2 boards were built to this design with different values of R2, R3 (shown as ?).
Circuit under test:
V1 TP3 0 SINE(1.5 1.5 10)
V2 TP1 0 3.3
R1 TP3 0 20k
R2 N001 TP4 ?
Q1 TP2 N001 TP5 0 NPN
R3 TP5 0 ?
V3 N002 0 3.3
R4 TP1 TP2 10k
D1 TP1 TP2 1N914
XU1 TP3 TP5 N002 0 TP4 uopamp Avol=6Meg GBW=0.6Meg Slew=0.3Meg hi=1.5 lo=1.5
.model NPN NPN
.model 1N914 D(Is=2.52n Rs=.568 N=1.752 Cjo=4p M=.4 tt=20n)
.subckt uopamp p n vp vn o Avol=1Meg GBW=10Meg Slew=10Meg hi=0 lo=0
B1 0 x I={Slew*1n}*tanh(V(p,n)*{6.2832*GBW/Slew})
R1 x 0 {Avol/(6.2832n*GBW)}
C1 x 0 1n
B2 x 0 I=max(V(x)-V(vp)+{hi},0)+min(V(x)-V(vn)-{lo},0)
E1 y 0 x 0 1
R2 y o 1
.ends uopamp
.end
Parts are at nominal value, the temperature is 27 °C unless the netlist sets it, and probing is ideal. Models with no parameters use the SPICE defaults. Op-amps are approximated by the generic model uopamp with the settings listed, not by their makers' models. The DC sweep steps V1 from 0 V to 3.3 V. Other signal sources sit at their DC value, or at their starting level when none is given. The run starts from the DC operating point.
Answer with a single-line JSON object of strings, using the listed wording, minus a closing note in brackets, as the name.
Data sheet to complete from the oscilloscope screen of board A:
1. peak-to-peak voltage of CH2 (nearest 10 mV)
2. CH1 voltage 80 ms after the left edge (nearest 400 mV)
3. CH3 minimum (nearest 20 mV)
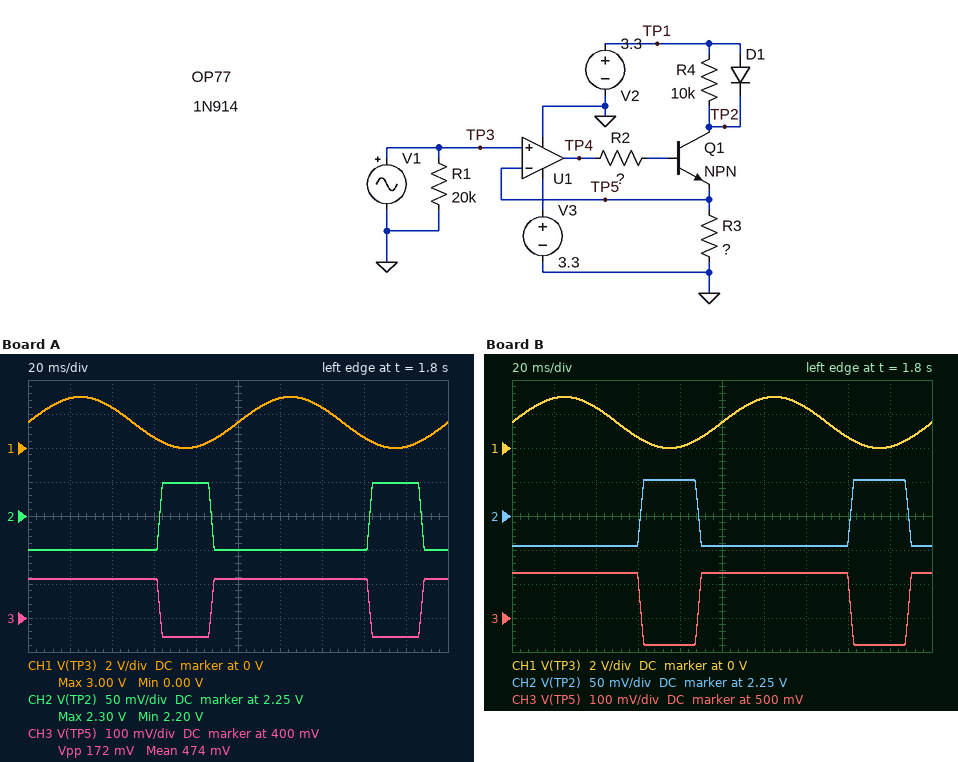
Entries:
{"peak-to-peak voltage of CH2": "100 mV", "CH1 voltage 80 ms after the left edge": "0 V", "CH3 minimum": "340 mV"}
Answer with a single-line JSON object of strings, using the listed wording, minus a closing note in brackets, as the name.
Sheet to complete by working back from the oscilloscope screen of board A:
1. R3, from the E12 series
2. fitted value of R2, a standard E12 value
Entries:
{"R3, from the E12 series": "1.2 Ω", "fitted value of R2, a standard E12 value": "82 Ω"}
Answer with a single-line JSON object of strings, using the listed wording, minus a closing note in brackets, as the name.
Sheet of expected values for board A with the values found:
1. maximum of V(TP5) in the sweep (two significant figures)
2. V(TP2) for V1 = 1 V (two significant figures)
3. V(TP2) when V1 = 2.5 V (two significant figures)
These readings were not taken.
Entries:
{"maximum of V(TP5) in the sweep": "520 mV", "V(TP2) for V1 = 1 V": "2.2 V", "V(TP2) when V1 = 2.5 V": "2.2 V"}
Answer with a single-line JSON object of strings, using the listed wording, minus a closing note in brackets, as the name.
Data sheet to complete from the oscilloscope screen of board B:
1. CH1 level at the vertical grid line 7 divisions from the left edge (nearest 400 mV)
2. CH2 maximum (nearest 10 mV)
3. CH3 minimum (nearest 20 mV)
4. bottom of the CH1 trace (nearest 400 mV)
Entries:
{"CH1 level at the vertical grid line 7 divisions from the left edge": "2.4 V", "CH2 maximum": "2.30 V", "CH3 minimum": "420 mV", "bottom of the CH1 trace": "0 V"}
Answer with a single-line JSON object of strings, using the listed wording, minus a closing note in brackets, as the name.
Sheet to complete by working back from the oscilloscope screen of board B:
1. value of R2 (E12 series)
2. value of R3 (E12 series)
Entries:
{"value of R2": "56 Ω", "value of R3": "1.5 Ω"}
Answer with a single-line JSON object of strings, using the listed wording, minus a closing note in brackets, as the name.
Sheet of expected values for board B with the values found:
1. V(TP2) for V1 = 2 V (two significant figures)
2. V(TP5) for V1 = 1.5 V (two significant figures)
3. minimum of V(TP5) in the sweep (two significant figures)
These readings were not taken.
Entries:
{"V(TP2) for V1 = 2 V": "2.2 V", "V(TP5) for V1 = 1.5 V": "630 mV", "minimum of V(TP5) in the sweep": "420 mV"}
